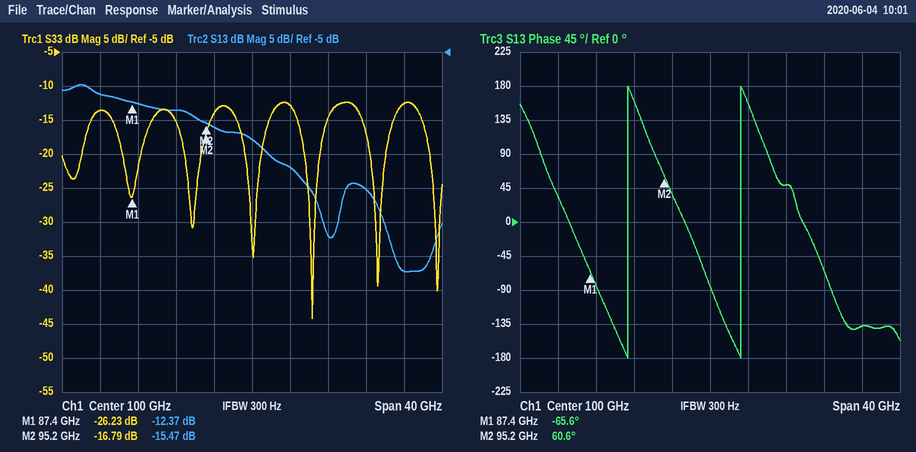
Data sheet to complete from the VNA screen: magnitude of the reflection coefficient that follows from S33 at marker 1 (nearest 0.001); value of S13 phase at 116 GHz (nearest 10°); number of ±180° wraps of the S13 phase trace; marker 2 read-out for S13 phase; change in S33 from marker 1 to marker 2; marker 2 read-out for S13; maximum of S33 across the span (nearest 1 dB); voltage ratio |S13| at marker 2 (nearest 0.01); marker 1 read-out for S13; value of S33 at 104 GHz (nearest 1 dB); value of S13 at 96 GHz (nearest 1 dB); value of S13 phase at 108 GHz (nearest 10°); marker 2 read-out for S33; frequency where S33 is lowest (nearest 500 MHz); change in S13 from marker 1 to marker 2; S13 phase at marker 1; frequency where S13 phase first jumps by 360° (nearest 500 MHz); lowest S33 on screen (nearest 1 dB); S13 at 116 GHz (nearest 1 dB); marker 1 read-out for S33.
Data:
0.049
-140°
2
60.6°
9.44 dB
-15.47 dB
-12 dB
0.17
-12.37 dB
-13 dB
-16 dB
50°
-16.79 dB
106.5 GHz
-3.10 dB
-65.6°
91.5 GHz
-44 dB
-37 dB
-26.23 dB
